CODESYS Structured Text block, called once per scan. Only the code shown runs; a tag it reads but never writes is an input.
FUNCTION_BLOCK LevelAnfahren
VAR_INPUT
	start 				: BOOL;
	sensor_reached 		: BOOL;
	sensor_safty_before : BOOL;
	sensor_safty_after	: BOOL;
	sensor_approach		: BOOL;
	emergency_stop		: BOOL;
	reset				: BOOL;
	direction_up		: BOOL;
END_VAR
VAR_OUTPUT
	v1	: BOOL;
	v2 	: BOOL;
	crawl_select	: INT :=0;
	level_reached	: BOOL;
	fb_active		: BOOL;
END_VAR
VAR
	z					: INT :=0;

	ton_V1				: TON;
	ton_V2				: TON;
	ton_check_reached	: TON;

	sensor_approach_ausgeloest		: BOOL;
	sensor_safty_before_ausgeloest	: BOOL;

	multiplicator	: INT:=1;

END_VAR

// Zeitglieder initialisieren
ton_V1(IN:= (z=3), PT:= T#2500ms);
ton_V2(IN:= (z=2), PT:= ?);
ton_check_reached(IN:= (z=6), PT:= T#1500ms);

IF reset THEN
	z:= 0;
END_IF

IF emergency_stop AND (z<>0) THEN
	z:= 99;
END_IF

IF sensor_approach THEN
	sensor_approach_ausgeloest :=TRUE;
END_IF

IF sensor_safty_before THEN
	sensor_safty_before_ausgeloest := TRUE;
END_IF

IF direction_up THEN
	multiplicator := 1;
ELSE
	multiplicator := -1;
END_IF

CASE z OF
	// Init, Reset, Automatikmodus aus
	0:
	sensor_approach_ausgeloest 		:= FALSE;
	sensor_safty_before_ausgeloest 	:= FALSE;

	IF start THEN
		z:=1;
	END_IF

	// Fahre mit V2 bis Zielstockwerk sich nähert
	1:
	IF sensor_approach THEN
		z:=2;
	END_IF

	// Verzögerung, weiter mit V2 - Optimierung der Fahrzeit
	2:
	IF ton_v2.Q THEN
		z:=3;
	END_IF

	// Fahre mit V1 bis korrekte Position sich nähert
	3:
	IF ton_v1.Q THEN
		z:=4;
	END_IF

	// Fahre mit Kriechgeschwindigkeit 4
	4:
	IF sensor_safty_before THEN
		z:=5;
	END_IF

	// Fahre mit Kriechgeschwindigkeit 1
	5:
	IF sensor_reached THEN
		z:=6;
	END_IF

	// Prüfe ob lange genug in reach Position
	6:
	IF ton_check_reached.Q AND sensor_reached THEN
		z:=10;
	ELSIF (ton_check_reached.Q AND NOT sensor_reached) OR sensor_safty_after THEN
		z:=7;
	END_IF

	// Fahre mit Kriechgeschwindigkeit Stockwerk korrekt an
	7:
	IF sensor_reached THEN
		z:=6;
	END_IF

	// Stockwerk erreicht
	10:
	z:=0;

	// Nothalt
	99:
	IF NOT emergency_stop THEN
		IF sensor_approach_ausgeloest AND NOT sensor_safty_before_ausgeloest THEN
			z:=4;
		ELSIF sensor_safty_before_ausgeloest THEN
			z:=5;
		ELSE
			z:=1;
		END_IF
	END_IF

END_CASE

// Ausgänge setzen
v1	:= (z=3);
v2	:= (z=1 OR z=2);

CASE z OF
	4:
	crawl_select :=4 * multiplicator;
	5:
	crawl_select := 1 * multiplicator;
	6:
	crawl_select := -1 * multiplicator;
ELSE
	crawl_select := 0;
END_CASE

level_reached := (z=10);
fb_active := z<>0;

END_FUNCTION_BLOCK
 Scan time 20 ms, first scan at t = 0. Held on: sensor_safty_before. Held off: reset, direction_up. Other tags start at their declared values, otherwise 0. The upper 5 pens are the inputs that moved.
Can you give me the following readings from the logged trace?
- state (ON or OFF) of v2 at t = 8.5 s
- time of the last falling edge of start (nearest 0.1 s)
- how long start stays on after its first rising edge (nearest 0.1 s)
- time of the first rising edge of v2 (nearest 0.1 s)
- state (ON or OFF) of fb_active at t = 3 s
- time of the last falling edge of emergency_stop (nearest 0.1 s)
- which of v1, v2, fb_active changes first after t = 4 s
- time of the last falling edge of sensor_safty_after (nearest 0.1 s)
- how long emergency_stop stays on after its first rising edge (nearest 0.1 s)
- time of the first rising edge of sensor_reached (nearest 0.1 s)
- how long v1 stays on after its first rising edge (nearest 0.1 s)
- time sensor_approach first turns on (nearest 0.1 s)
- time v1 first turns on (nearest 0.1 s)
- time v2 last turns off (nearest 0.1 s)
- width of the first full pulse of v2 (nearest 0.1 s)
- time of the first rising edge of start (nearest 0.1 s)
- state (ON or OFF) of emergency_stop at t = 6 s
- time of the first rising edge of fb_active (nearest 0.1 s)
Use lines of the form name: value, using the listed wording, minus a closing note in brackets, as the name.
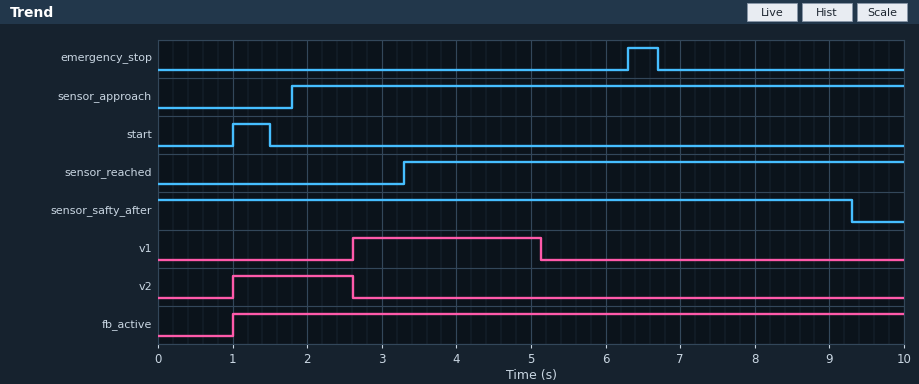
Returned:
state (ON or OFF) of v2 at t = 8.5 s: OFF
time of the last falling edge of start: 1.5 s
how long start stays on after its first rising edge: 0.5 s
time of the first rising edge of v2: 1.0 s
state (ON or OFF) of fb_active at t = 3 s: ON
time of the last falling edge of emergency_stop: 6.7 s
which of v1, v2, fb_active changes first after t = 4 s: v1
time of the last falling edge of sensor_safty_after: 9.3 s
how long emergency_stop stays on after its first rising edge: 0.4 s
time of the first rising edge of sensor_reached: 3.3 s
how long v1 stays on after its first rising edge: 2.5 s
time sensor_approach first turns on: 1.8 s
time v1 first turns on: 2.6 s
time v2 last turns off: 2.6 s
width of the first full pulse of v2: 1.6 s
time of the first rising edge of start: 1.0 s
state (ON or OFF) of emergency_stop at t = 6 s: OFF
time of the first rising edge of fb_active: 1.0 s
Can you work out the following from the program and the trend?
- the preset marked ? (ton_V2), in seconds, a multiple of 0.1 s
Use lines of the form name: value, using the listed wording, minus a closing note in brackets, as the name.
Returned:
the preset marked ? (ton_V2), in seconds, a multiple of 0.1 s: 0.8 s
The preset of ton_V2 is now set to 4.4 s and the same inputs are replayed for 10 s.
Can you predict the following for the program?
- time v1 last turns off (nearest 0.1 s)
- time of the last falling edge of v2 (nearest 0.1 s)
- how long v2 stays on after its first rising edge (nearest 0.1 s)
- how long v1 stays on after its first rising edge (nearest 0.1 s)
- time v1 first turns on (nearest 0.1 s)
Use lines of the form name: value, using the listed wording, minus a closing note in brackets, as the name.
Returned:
time v1 last turns off: 6.3 s
time of the last falling edge of v2: 6.2 s
how long v2 stays on after its first rising edge: 5.2 s
how long v1 stays on after its first rising edge: 0.1 s
time v1 first turns on: 6.2 s
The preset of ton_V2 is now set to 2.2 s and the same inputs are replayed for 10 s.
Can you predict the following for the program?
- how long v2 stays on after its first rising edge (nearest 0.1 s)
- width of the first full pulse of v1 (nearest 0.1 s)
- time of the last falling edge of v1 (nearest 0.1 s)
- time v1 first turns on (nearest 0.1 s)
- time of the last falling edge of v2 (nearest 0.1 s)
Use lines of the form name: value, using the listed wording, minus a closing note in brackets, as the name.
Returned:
how long v2 stays on after its first rising edge: 3.0 s
width of the first full pulse of v1: 2.3 s
time of the last falling edge of v1: 6.3 s
time v1 first turns on: 4.0 s
time of the last falling edge of v2: 4.0 s
